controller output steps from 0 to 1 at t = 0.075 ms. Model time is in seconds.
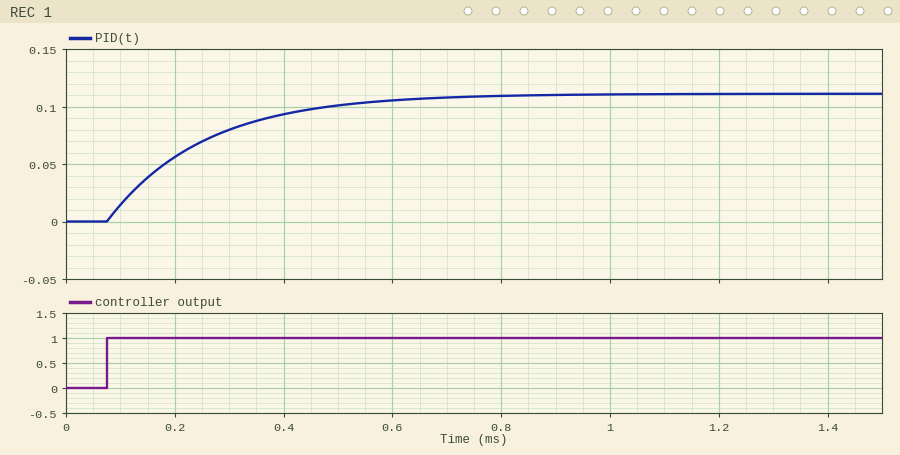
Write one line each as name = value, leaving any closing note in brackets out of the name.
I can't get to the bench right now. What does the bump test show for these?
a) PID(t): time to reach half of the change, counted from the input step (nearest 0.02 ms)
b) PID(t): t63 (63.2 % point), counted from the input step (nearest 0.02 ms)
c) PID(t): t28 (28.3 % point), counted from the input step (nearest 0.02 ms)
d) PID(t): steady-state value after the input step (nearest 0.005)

PID(t): time to reach half of the change, counted from the input step = 0.12 ms
PID(t): t63 (63.2 % point), counted from the input step = 0.18 ms
PID(t): t28 (28.3 % point), counted from the input step = 0.06 ms
PID(t): steady-state value after the input step = 0.110
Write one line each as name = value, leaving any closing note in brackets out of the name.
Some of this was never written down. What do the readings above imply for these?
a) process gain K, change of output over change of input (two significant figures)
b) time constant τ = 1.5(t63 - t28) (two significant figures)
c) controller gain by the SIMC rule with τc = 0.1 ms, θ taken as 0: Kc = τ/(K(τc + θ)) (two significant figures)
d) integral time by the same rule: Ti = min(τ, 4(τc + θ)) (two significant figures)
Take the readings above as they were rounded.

process gain K, change of output over change of input = 0.11
time constant τ = 1.5(t63 - t28) = 0.18 ms
controller gain by the SIMC rule with τc = 0.1 ms, θ taken as 0: Kc = τ/(K(τc + θ)) = 16
integral time by the same rule: Ti = min(τ, 4(τc + θ)) = 0.18 ms
